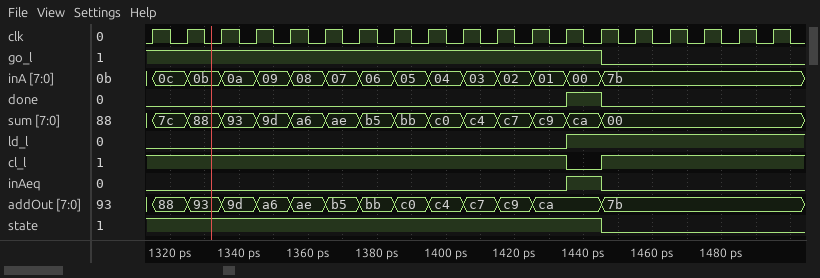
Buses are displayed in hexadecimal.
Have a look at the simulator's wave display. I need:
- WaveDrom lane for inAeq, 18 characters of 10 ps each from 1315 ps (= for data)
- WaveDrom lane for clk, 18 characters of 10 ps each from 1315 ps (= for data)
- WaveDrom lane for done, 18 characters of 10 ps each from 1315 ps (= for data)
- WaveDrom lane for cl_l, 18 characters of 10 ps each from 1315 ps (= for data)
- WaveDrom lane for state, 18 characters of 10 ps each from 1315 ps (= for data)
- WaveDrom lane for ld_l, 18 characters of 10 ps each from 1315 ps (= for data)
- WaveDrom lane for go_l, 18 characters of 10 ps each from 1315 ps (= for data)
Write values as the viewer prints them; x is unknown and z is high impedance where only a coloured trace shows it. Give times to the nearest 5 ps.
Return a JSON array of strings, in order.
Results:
["{name: 'inAeq', wave: '0...........10....'}", "{name: 'clk', wave: 'p.................'}", "{name: 'done', wave: '0...........10....'}", "{name: 'cl_l', wave: '1...........01....'}", "{name: 'state', wave: '1............0....'}", "{name: 'ld_l', wave: '0...........1.....'}", "{name: 'go_l', wave: '1............0....'}"]
